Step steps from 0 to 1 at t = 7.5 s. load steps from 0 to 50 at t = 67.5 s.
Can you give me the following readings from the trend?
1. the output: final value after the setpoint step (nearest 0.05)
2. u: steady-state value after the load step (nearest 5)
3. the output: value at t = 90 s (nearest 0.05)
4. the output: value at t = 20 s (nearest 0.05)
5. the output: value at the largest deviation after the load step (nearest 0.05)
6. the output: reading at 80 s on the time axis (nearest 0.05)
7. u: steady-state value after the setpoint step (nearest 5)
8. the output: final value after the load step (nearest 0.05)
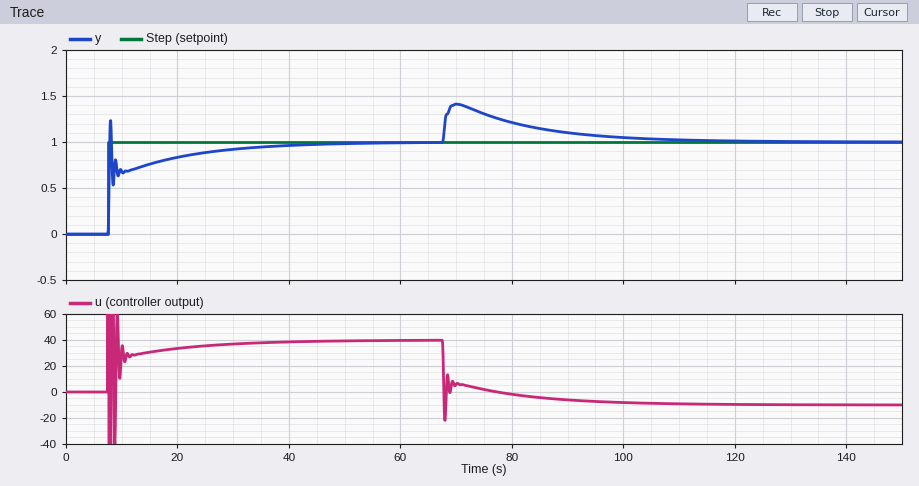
1.00
-10
1.10
0.85
1.40
1.20
40
1.00
